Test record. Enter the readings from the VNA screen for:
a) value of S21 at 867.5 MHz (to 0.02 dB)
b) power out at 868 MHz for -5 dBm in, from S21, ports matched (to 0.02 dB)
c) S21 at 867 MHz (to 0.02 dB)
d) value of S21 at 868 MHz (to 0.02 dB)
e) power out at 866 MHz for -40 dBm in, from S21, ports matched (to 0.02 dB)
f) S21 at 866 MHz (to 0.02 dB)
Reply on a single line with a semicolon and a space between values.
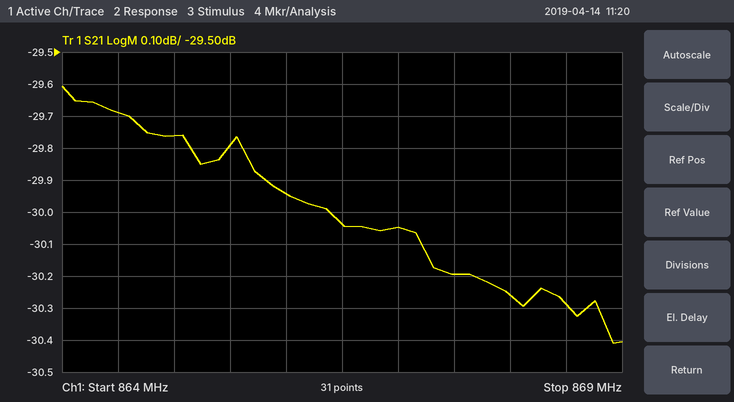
-30.20 dB; -35.26 dBm; -30.04 dB; -30.26 dB; -69.94 dBm; -29.94 dB
